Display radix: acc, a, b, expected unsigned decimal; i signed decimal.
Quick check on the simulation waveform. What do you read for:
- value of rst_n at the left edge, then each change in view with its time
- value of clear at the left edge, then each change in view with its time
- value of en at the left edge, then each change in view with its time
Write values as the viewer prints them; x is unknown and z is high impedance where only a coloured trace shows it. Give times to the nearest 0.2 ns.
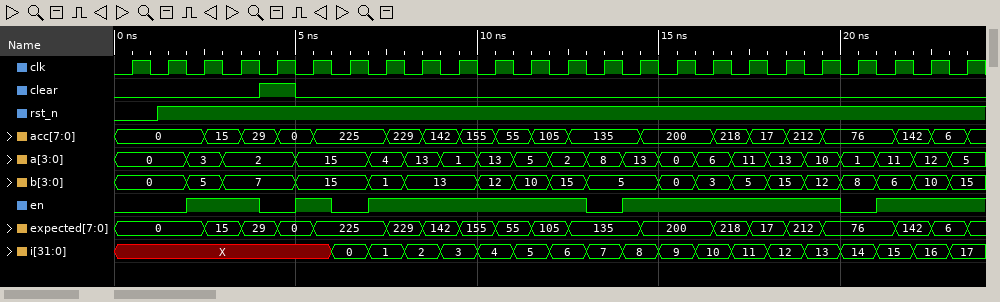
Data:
0, 1 at 1.2 ns
0, 1 at 4 ns, 0 at 5 ns
0, 1 at 2 ns, 0 at 4 ns, 1 at 5 ns, 0 at 6 ns, 1 at 7 ns, 0 at 13 ns, 1 at 14 ns, 0 at 20 ns, 1 at 21 ns
